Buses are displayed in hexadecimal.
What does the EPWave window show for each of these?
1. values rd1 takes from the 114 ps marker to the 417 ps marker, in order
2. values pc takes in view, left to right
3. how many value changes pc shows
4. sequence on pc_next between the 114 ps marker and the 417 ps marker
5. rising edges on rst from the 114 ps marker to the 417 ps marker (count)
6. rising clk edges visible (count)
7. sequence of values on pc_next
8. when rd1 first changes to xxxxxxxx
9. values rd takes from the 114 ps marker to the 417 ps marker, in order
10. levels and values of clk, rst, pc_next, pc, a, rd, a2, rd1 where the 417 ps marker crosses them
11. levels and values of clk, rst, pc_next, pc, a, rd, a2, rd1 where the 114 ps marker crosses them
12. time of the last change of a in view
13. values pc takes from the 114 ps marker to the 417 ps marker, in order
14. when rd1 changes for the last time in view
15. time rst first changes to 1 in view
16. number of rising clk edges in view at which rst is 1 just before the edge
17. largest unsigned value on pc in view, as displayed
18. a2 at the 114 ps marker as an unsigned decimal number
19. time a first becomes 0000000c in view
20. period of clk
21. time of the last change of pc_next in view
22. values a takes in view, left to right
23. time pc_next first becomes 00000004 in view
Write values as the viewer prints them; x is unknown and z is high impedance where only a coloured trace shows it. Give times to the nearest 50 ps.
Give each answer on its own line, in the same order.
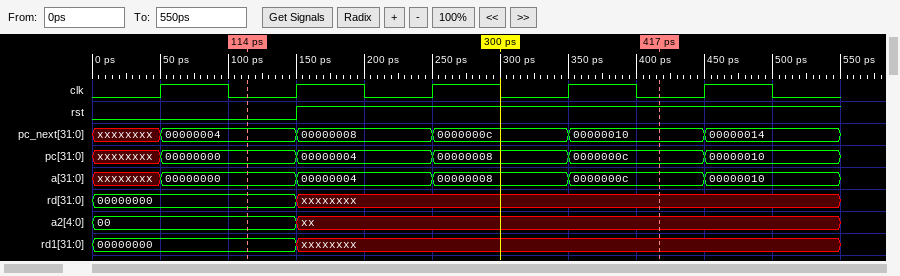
00000000, xxxxxxxx
xxxxxxxx, 00000000, 00000004, 00000008, 0000000c, 00000010
5
00000004, 00000008, 0000000c, 00000010
1
5
xxxxxxxx, 00000004, 00000008, 0000000c, 00000010, 00000014
150 ps
00000000, xxxxxxxx
clk=0, rst=1, pc_next=00000010, pc=0000000c, a=0000000c, rd=xxxxxxxx, a2=xx, rd1=xxxxxxxx
clk=0, rst=0, pc_next=00000004, pc=00000000, a=00000000, rd=00000000, a2=00, rd1=00000000
450 ps
00000000, 00000004, 00000008, 0000000c
150 ps
150 ps
3
00000010
0
350 ps
100 ps
450 ps
xxxxxxxx, 00000000, 00000004, 00000008, 0000000c, 00000010
50 ps
